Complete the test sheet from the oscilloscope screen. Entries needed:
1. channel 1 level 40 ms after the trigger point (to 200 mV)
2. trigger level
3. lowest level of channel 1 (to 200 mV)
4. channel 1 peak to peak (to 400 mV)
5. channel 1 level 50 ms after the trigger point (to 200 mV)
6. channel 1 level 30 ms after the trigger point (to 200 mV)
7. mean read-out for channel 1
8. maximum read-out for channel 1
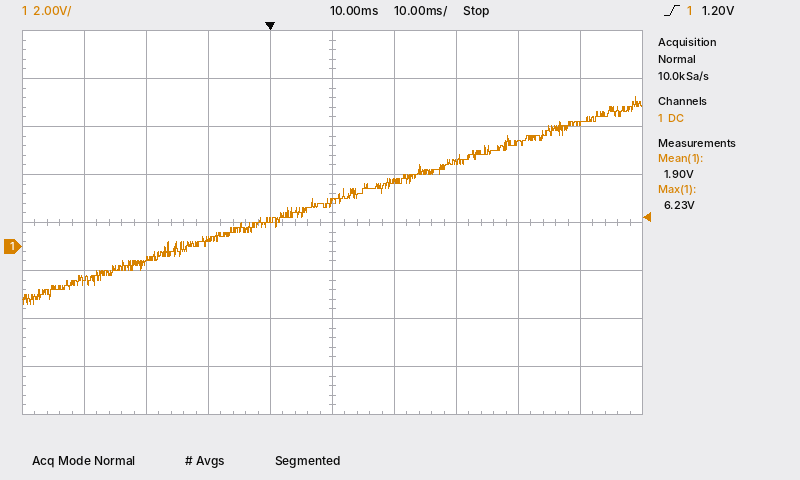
4.4 V
1.20 V
-2.4 V
8.8 V
5.2 V
3.6 V
1.90 V
6.23 V
